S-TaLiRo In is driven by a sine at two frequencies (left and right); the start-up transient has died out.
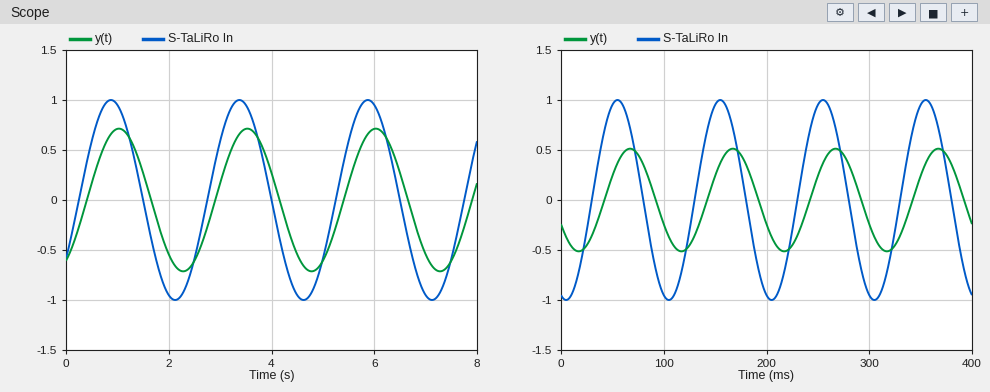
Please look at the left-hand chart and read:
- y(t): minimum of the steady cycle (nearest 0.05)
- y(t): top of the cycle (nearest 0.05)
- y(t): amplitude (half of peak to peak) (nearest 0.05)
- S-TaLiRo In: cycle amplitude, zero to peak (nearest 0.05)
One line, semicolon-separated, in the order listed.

-0.70; 0.70; 0.70; 1.00
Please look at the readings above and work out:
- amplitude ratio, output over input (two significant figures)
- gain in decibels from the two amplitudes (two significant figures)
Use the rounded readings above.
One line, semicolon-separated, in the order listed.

0.70; -3.1 dB
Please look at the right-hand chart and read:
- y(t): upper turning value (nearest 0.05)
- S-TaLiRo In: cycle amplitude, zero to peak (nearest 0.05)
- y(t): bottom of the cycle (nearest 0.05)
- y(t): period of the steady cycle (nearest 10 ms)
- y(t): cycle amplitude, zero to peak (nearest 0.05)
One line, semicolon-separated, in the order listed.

0.50; 1.00; -0.50; 100 ms; 0.50
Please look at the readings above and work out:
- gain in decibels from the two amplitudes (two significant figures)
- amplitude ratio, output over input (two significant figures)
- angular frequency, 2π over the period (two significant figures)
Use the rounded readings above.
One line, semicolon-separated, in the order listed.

-6.0 dB; 0.50; 0.063 rad/ms
